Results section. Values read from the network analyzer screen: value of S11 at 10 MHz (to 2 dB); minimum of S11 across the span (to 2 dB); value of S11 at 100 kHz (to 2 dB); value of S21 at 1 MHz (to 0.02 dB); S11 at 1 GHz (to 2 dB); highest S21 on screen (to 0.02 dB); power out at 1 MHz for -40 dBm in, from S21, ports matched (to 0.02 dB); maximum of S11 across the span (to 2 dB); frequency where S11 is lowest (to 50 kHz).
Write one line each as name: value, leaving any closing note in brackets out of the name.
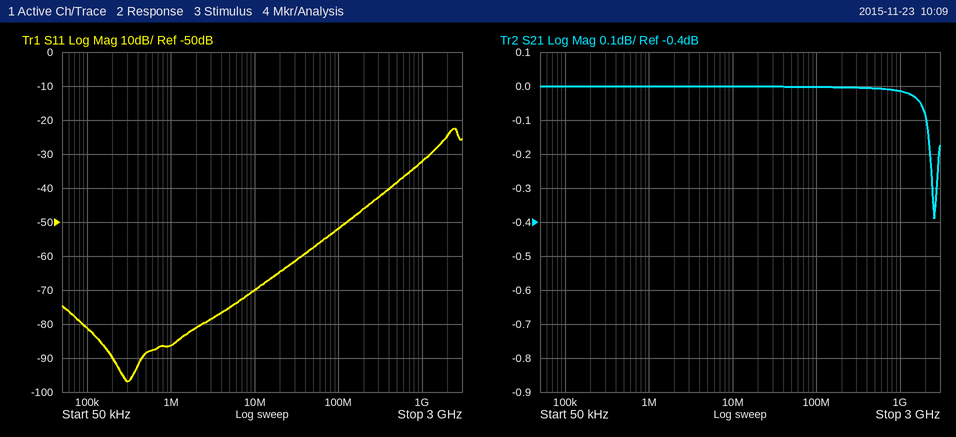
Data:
value of S11 at 10 MHz: -70 dB
minimum of S11 across the span: -96 dB
value of S11 at 100 kHz: -82 dB
value of S21 at 1 MHz: 0.00 dB
S11 at 1 GHz: -32 dB
highest S21 on screen: 0.00 dB
power out at 1 MHz for -40 dBm in, from S21, ports matched: -40.00 dBm
maximum of S11 across the span: -22 dB
frequency where S11 is lowest: 300 kHz
